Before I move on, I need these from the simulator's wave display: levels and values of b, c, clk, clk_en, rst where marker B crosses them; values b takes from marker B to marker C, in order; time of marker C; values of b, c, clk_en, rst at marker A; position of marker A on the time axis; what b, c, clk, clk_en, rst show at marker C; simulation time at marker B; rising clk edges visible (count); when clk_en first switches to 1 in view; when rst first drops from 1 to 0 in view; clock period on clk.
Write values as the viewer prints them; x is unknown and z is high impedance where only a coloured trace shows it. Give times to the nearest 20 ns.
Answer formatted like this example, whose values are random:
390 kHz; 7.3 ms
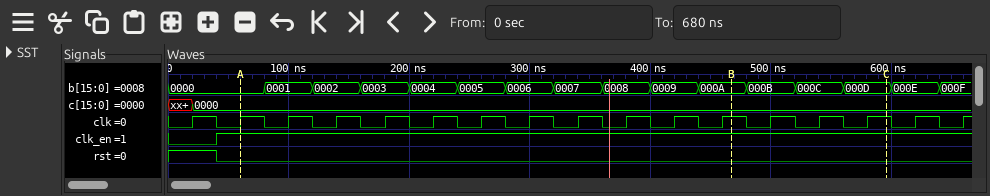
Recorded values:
b=000A, c=0000, clk=1, clk_en=1, rst=0; 000A, 000B, 000C, 000D; 600 ns; b=0000, c=0000, clk_en=1, rst=0; 60 ns; b=000D, c=0000, clk=1, clk_en=1, rst=0; 460 ns; 17; 40 ns; 40 ns; 40 ns
